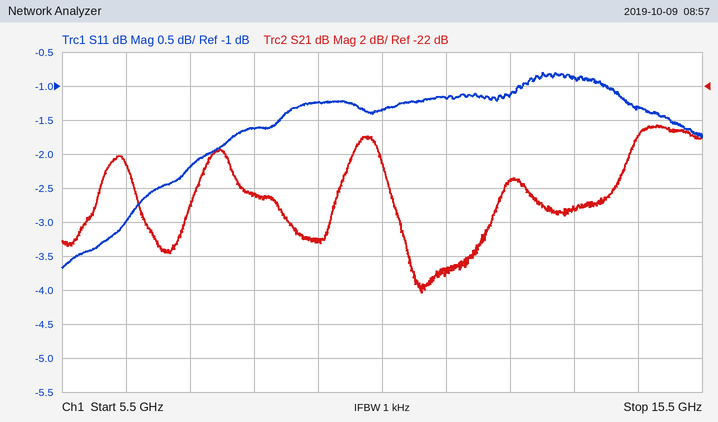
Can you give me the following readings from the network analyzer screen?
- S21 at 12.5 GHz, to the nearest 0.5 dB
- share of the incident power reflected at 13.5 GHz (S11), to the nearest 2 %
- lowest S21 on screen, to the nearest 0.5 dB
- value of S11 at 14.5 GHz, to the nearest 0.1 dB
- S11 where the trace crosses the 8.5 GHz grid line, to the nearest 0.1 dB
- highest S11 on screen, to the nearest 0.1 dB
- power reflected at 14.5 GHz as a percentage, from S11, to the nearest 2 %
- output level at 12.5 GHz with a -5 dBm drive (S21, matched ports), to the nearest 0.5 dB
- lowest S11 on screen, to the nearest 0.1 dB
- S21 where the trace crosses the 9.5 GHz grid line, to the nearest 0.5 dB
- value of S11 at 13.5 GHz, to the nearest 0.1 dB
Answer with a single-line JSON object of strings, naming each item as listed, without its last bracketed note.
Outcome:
{"S21 at 12.5 GHz, to the nearest 0.5 dB": "-27.5 dB", "share of the incident power reflected at 13.5 GHz (S11), to the nearest 2 %": "82 %", "lowest S21 on screen, to the nearest 0.5 dB": "-34.0 dB", "value of S11 at 14.5 GHz, to the nearest 0.1 dB": "-1.3 dB", "S11 where the trace crosses the 8.5 GHz grid line, to the nearest 0.1 dB": "-1.6 dB", "highest S11 on screen, to the nearest 0.1 dB": "-0.8 dB", "power reflected at 14.5 GHz as a percentage, from S11, to the nearest 2 %": "74 %", "output level at 12.5 GHz with a -5 dBm drive (S21, matched ports), to the nearest 0.5 dB": "-32.5 dBm", "lowest S11 on screen, to the nearest 0.1 dB": "-3.7 dB", "S21 where the trace crosses the 9.5 GHz grid line, to the nearest 0.5 dB": "-31.0 dB", "value of S11 at 13.5 GHz, to the nearest 0.1 dB": "-0.9 dB"}
